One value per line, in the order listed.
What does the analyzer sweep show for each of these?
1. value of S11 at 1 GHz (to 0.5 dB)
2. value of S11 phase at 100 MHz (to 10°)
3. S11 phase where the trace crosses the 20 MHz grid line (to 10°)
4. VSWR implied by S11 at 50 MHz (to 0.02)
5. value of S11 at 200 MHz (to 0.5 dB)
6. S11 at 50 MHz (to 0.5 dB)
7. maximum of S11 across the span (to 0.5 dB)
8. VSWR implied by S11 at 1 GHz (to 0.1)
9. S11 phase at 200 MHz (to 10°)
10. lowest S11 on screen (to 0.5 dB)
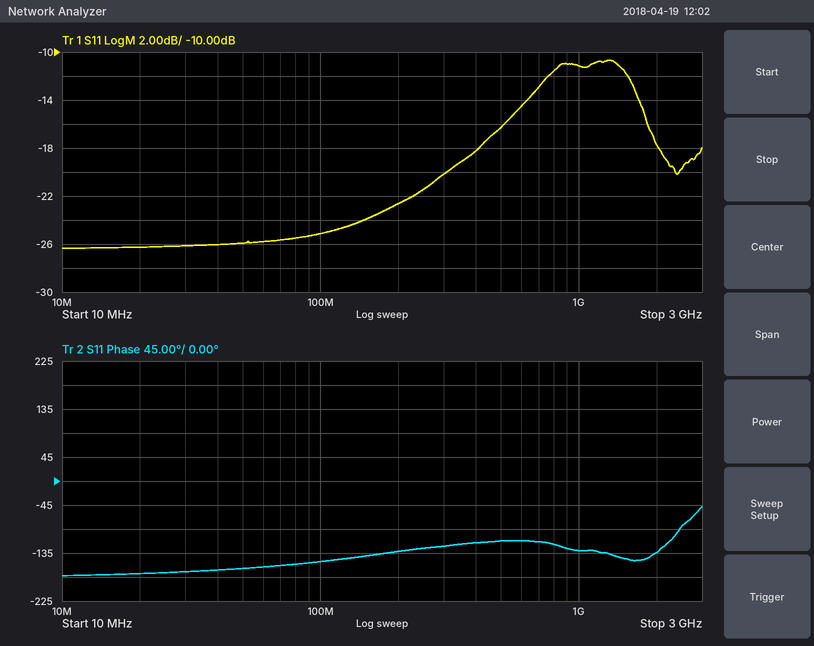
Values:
-11.0 dB
-150°
-170°
1.10
-22.5 dB
-26.0 dB
-10.5 dB
1.8
-130°
-26.5 dB
